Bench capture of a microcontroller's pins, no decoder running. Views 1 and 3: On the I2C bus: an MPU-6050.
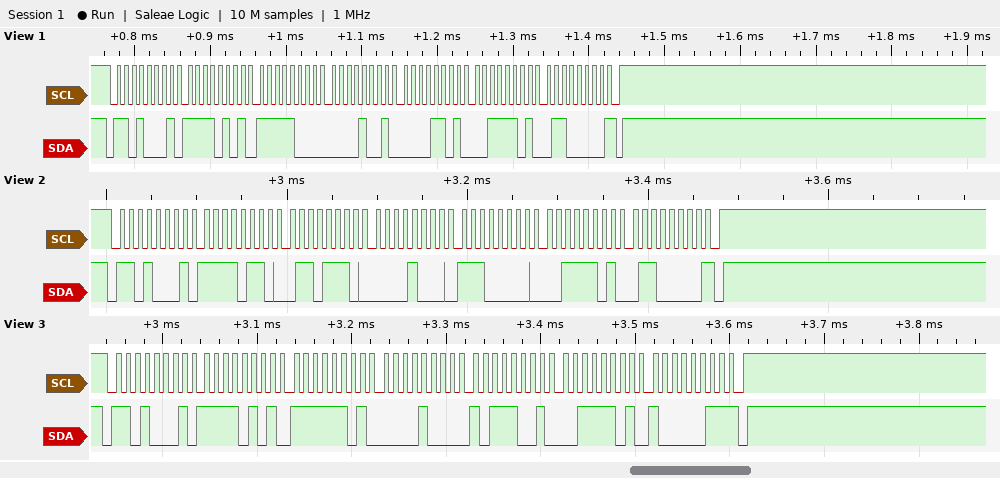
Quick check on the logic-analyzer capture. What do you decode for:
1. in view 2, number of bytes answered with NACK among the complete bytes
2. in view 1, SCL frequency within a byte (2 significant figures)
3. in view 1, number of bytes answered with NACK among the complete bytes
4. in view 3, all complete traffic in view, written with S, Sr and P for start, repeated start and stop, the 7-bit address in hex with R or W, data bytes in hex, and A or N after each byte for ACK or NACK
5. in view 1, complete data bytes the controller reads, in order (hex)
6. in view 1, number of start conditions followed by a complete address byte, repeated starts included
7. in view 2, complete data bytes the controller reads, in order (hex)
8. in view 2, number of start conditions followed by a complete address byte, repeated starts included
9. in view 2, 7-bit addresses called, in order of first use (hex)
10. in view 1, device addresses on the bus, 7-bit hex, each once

1
100 kHz
1
S 68R A F5 A FD A 08 A B9 A 3D A 83 N P
F5 F8 09 0D 3D 60
1
F6 6E 08 E0 3D 60
1
0x68
0x68
